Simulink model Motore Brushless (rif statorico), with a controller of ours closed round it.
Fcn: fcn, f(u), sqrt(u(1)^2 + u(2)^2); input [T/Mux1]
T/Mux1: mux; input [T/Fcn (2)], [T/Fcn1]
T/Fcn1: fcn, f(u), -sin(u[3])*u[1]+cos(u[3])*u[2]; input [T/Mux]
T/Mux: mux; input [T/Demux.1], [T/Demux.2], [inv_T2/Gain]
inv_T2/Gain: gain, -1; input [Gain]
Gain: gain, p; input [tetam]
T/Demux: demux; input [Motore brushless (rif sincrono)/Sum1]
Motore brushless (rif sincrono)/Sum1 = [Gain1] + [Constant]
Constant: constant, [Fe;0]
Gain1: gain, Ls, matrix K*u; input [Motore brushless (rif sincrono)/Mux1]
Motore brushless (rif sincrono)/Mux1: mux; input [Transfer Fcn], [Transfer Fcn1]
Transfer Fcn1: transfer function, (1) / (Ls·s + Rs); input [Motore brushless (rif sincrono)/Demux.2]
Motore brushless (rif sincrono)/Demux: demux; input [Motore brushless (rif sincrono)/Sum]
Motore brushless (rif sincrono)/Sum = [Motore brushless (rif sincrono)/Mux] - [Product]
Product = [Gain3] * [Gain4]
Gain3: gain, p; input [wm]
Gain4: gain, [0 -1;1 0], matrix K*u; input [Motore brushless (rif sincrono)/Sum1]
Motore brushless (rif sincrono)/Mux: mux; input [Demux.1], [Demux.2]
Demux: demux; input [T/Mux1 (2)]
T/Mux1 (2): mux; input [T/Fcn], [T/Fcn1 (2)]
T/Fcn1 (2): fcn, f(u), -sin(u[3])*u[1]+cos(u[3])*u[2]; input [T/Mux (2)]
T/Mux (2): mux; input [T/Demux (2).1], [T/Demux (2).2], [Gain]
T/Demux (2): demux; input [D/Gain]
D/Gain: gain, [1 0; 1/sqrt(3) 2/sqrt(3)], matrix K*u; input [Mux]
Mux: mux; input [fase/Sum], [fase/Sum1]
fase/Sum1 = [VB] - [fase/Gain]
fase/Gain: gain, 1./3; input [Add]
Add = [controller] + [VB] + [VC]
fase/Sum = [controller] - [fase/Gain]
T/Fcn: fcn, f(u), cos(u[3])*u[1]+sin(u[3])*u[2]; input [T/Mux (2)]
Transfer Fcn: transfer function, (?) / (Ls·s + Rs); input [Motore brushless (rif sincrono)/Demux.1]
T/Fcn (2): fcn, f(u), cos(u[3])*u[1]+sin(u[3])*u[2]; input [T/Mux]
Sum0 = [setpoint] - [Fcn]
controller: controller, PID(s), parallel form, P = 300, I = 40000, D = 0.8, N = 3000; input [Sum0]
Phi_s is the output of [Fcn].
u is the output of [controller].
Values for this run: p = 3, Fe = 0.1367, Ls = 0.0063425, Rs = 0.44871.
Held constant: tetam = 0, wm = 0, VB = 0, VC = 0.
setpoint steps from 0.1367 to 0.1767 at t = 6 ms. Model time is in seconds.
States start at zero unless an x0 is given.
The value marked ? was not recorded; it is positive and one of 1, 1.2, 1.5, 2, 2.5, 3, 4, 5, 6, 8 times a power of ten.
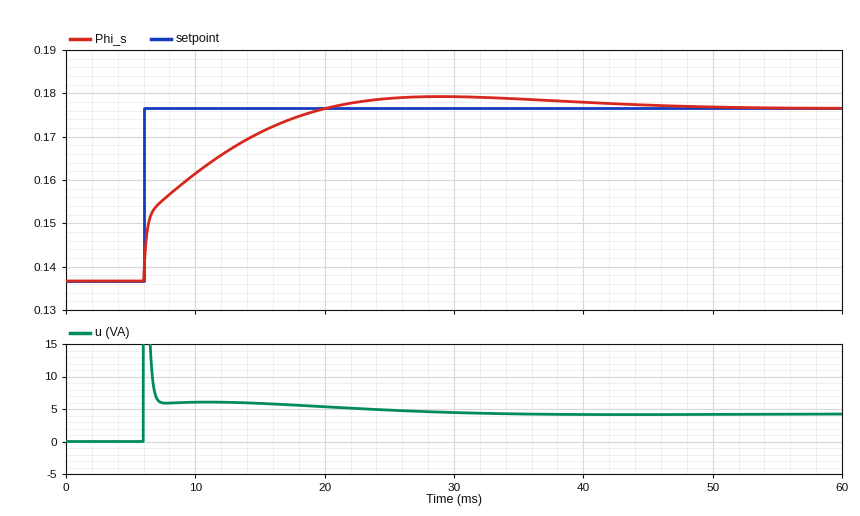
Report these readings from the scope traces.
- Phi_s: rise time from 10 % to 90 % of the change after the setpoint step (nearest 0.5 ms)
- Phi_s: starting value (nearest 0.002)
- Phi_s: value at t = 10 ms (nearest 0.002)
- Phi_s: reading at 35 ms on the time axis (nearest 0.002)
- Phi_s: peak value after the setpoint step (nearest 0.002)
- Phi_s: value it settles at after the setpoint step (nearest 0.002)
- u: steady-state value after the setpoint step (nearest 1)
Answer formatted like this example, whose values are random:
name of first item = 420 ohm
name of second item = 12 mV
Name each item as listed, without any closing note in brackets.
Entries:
Phi_s: rise time from 10 % to 90 % of the change after the setpoint step = 10.0 ms
Phi_s: starting value = 0.136
Phi_s: value at t = 10 ms = 0.162
Phi_s: reading at 35 ms on the time axis = 0.178
Phi_s: peak value after the setpoint step = 0.180
Phi_s: value it settles at after the setpoint step = 0.176
u: steady-state value after the setpoint step = 4
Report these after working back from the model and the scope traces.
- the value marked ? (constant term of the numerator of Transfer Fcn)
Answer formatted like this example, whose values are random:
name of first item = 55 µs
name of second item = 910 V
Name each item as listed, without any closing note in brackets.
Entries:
the value marked ? = 1
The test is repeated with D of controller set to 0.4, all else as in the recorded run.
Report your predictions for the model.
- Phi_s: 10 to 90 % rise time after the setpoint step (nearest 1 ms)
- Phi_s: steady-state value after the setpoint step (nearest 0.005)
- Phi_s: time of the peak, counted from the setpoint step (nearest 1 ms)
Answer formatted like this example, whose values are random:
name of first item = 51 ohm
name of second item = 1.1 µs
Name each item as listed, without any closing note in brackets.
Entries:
Phi_s: 10 to 90 % rise time after the setpoint step = 9 ms
Phi_s: steady-state value after the setpoint step = 0.175
Phi_s: time of the peak, counted from the setpoint step = 20 ms
